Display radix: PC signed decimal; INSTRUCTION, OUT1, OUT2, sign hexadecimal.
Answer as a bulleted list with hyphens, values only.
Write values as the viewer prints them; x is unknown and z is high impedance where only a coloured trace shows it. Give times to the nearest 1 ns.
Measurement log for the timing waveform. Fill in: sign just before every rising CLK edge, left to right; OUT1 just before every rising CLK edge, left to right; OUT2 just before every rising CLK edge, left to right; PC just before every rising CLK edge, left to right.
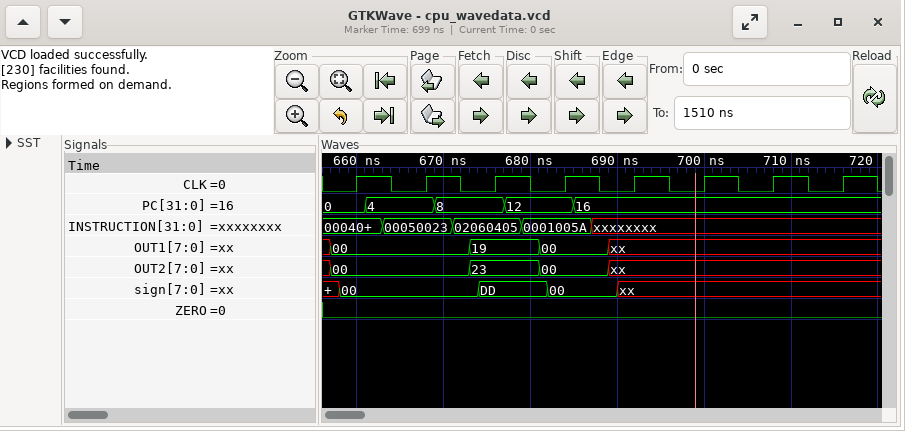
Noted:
- 00, 00, DD, 00, xx, xx, xx, xx
- 00, 00, 19, 00, xx, xx, xx, xx
- 00, 00, 23, 00, xx, xx, xx, xx
- 0, 4, 8, 12, 16, 16, 16, 16
